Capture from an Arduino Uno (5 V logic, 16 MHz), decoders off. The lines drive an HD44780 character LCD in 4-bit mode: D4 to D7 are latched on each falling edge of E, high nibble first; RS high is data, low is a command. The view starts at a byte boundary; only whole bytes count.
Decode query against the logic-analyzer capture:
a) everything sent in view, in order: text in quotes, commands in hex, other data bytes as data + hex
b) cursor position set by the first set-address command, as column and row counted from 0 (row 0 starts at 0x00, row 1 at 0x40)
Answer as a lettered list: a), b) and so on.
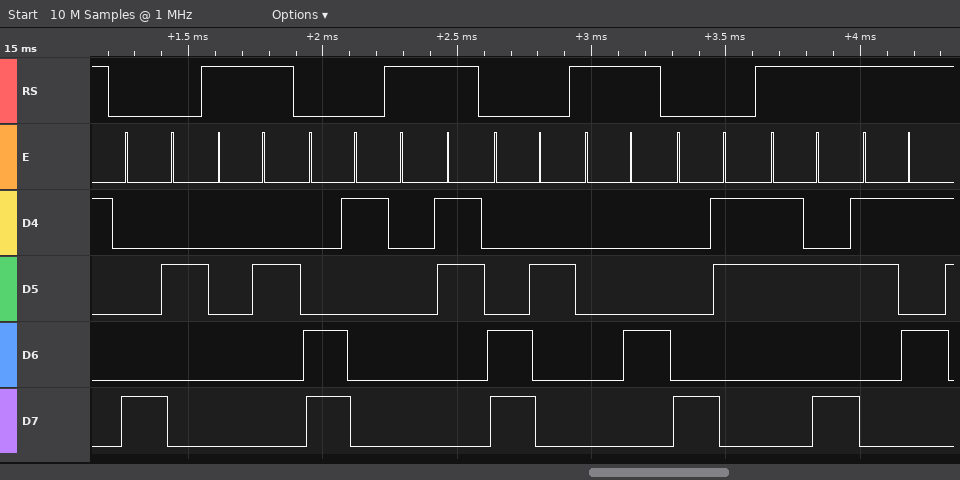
a) 0x82 data 02 0xC1 data 03 0xC2 data 04 0x83 ":5"
b) column 2, row 0
